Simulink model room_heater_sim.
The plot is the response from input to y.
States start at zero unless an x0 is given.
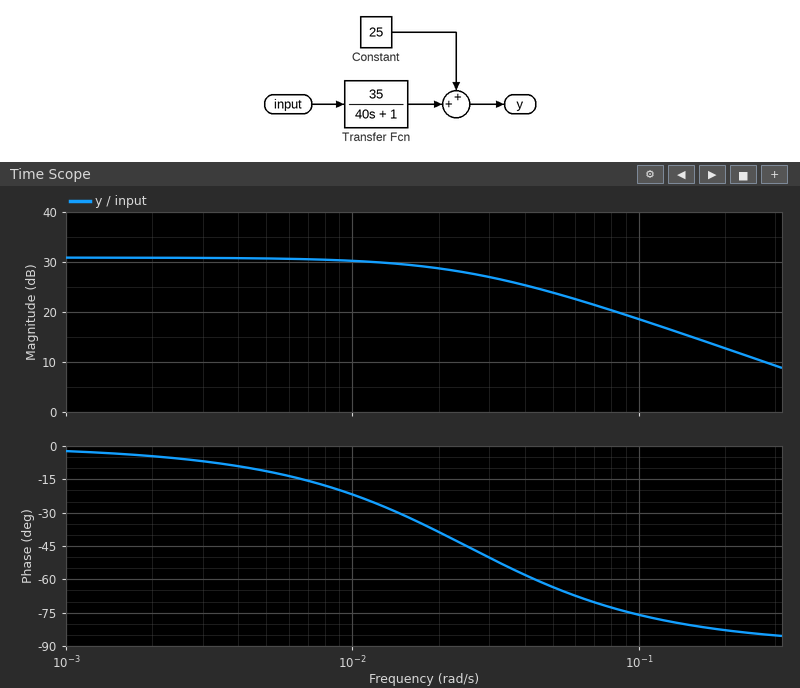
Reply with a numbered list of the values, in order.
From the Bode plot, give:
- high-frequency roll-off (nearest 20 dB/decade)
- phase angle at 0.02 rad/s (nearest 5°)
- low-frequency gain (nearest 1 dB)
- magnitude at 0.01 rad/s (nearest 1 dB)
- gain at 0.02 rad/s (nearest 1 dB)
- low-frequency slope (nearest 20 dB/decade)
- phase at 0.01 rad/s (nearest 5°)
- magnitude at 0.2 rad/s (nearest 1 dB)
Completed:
1. -20 dB/decade
2. -40°
3. 31 dB
4. 30 dB
5. 29 dB
6. 0 dB/decade
7. -20°
8. 13 dB
